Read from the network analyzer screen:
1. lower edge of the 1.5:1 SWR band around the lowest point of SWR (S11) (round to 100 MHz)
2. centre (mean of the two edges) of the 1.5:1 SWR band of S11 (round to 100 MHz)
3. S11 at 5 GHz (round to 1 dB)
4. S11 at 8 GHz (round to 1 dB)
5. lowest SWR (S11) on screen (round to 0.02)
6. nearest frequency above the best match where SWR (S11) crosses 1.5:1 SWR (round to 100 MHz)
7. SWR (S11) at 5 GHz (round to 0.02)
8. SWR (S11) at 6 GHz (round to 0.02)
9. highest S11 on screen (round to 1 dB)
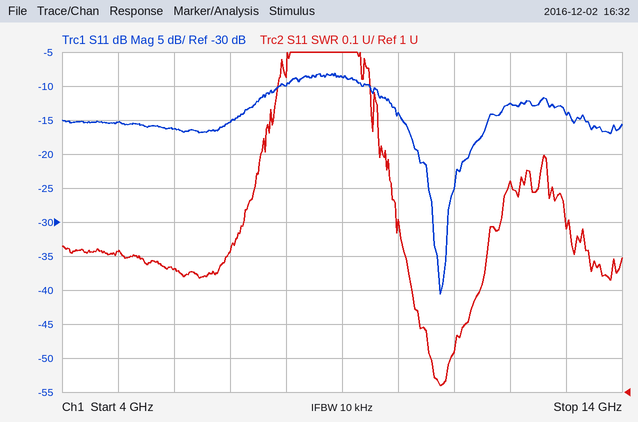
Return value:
10.0 GHz
10.9 GHz
-15 dB
-10 dB
1.02
11.8 GHz
1.42
1.36
-8 dB
